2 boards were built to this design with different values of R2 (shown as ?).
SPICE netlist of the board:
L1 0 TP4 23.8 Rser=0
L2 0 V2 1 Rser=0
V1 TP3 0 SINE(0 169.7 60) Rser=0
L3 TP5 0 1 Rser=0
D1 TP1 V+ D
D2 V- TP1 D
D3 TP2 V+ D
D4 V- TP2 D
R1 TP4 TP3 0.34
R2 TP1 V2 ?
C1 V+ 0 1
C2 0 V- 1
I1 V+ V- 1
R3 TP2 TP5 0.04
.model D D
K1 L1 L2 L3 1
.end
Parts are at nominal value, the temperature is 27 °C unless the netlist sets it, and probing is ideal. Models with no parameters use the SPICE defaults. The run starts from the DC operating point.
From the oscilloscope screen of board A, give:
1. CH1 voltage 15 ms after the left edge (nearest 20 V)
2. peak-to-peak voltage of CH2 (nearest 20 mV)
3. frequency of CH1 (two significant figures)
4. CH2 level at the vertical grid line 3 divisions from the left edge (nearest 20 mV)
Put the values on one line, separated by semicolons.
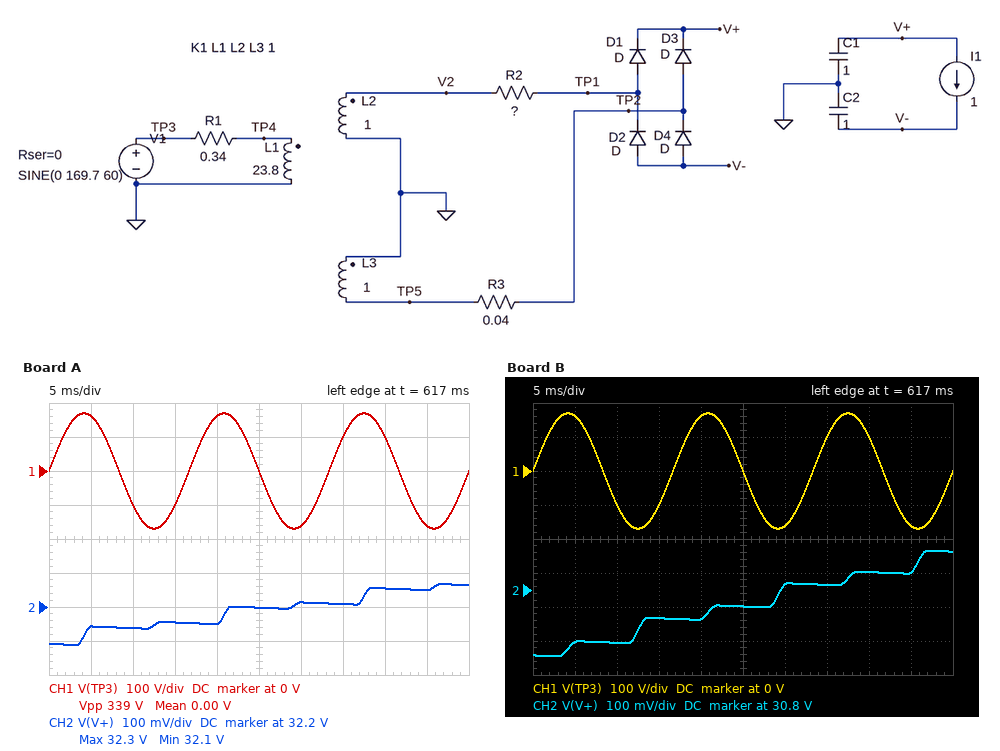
-100 V; 180 mV; 60 Hz; 32.16 V
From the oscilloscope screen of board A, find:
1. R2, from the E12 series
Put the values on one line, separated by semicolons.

0.015 Ω
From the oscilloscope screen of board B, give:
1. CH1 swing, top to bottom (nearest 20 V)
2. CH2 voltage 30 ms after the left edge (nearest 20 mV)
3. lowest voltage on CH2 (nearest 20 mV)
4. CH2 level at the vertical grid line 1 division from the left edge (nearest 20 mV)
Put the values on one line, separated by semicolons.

340 V; 30.82 V; 30.60 V; 30.64 V
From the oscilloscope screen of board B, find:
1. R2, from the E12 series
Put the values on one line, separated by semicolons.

0.068 Ω
